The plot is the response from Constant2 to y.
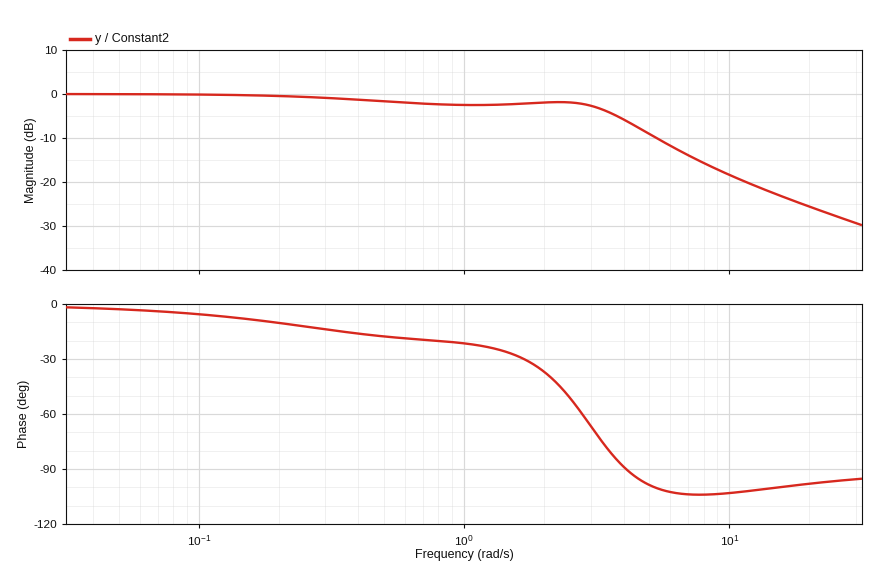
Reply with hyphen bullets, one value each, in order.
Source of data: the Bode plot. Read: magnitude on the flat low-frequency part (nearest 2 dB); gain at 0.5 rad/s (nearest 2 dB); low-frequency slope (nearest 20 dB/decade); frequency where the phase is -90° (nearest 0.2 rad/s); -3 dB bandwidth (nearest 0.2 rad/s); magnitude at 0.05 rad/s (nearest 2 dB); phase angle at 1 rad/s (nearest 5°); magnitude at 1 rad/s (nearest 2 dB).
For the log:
- 0 dB
- -2 dB
- 0 dB/decade
- 4.0 rad/s
- 3.2 rad/s
- 0 dB
- -20°
- -2 dB
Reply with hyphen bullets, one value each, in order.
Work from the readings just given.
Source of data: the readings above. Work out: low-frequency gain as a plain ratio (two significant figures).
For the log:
- 1.0
